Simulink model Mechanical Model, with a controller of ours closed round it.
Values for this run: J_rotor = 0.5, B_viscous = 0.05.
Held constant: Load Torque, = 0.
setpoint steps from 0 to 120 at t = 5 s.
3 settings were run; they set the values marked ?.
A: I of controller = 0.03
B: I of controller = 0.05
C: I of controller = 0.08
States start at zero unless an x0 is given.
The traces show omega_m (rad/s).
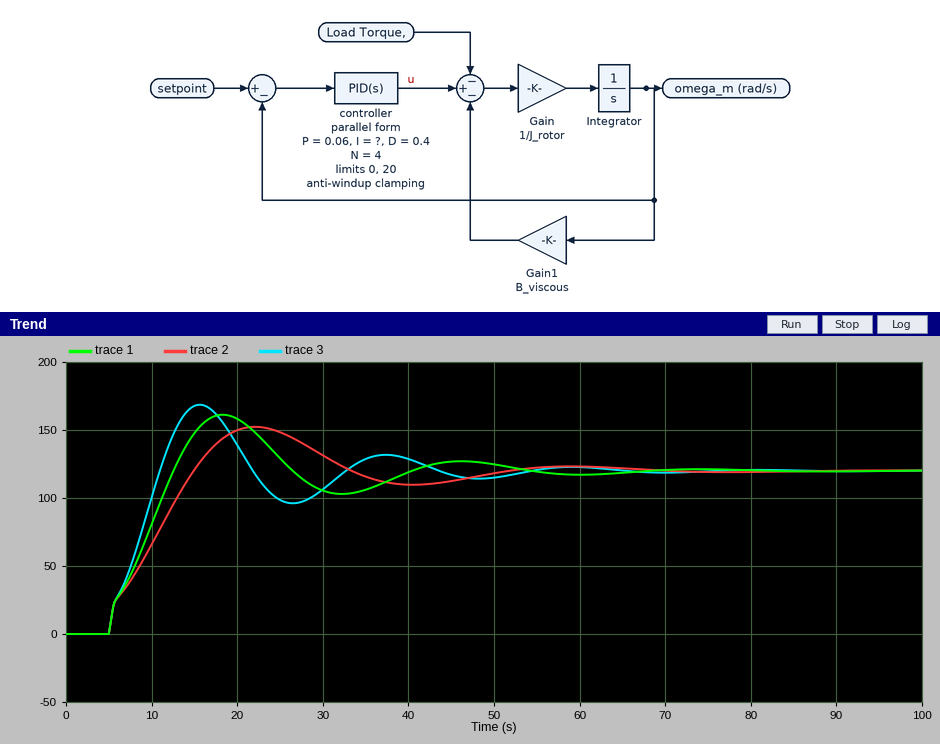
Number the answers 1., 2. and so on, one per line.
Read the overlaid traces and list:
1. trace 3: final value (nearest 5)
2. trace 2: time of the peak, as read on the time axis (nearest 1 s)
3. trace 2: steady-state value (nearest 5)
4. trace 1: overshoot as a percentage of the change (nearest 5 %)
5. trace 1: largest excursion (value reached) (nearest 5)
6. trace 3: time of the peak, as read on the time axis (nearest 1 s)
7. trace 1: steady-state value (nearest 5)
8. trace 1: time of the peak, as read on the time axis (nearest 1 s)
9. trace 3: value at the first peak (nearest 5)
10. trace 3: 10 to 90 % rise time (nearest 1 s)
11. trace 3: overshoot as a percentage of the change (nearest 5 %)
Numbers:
1. 120
2. 22 s
3. 120
4. 35 %
5. 160
6. 16 s
7. 120
8. 18 s
9. 170
10. 5 s
11. 40 %
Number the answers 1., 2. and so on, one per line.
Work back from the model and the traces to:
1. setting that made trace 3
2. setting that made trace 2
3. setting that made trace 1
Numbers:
1. C
2. A
3. B
